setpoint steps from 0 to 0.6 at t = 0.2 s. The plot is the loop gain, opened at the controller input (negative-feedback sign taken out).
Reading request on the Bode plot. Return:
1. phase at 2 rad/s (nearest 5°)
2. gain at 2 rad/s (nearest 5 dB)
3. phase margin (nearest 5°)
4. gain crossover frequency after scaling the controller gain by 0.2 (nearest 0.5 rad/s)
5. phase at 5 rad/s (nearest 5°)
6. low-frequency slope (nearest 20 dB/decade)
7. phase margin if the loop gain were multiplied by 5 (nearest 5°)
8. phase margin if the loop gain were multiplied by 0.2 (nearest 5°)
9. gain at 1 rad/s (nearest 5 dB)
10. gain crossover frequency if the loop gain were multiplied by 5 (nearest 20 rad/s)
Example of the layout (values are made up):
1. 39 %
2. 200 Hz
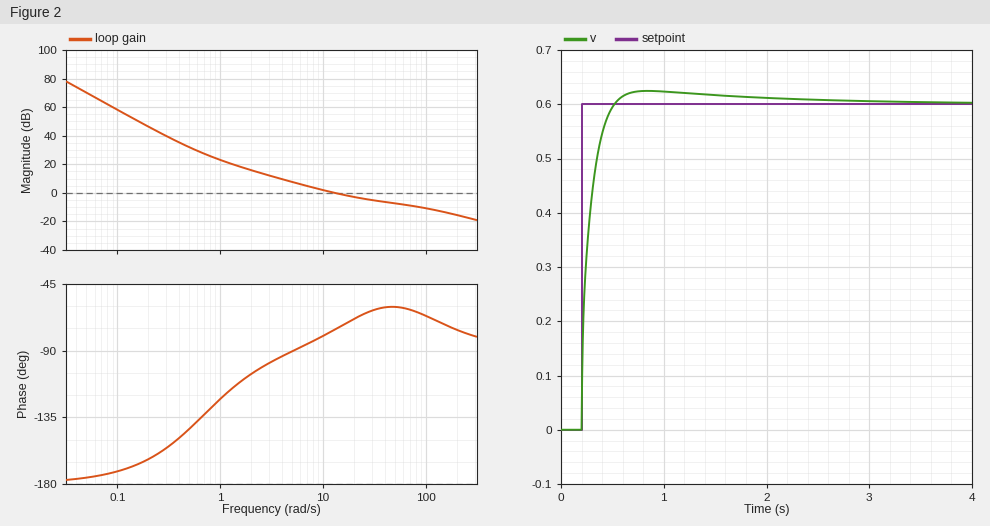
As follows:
1. -105°
2. 15 dB
3. 105°
4. 2.5 rad/s
5. -90°
6. -40 dB/decade
7. 105°
8. 80°
9. 25 dB
10. 160 rad/s
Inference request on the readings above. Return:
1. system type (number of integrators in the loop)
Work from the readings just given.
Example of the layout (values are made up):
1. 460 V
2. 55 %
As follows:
1. 2
